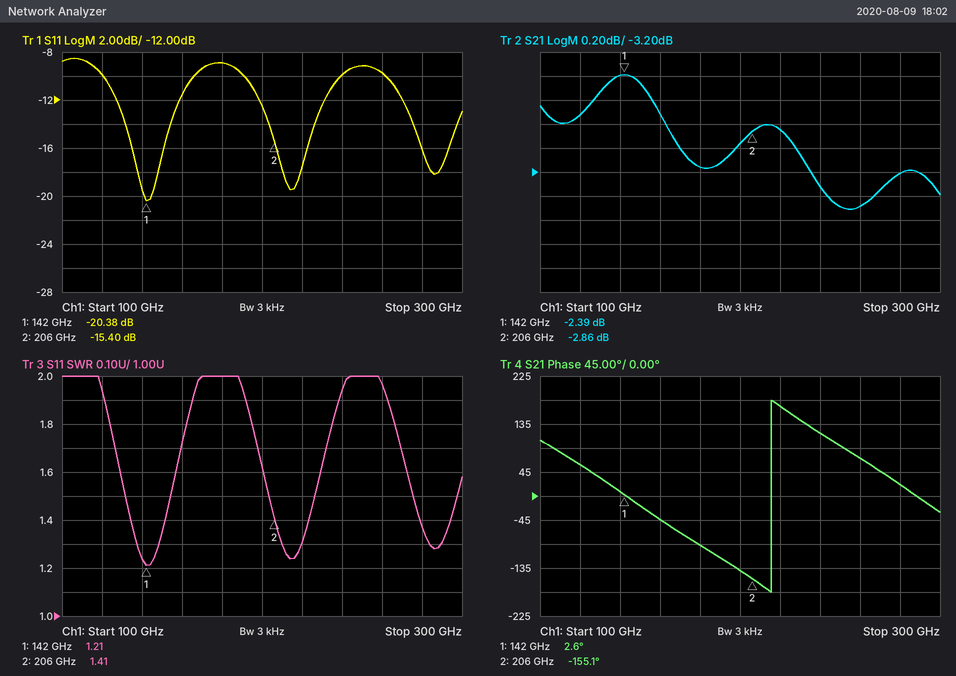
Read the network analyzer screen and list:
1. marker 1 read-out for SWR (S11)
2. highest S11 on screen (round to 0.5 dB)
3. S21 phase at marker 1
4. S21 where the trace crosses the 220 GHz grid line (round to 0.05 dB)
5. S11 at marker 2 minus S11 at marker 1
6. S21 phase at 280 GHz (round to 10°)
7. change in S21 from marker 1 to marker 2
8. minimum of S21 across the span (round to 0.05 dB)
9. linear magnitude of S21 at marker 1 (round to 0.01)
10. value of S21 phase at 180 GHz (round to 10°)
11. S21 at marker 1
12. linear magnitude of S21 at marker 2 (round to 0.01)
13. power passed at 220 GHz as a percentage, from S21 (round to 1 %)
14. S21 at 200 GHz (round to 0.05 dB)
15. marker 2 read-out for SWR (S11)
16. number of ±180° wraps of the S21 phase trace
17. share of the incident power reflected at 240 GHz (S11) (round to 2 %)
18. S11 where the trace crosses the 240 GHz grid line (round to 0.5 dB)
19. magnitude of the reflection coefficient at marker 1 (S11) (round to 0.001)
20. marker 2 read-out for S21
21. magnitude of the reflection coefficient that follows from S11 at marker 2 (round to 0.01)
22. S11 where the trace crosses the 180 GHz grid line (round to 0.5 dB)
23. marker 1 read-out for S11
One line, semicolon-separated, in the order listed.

1.21; -8.5 dB; 2.6°; -2.85 dB; 4.98 dB; 20°; -0.47 dB; -3.50 dB; 0.76; -90°; -2.39 dB; 0.72; 52 %; -2.95 dB; 1.41; 1; 10 %; -10.0 dB; 0.096; -2.86 dB; 0.17; -9.0 dB; -20.38 dB
